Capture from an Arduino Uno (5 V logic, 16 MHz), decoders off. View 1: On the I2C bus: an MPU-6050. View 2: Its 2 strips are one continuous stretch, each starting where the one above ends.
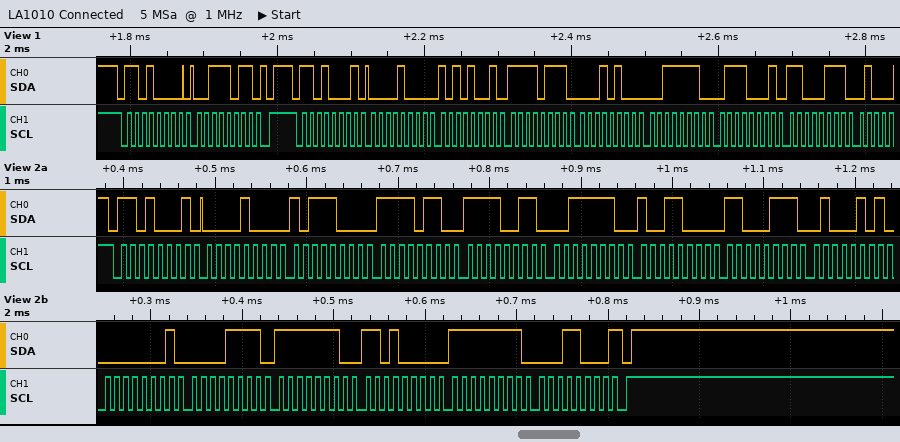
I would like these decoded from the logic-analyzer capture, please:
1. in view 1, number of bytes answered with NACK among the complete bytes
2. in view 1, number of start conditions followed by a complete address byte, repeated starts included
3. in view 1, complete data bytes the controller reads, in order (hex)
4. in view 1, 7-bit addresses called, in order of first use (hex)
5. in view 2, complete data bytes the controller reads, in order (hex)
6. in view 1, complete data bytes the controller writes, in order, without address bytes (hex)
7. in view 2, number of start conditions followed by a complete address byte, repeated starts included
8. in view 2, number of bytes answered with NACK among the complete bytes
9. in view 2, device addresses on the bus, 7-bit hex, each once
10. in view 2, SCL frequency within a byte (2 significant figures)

0
2
08 A9 F7 14 3E 71 C7
0x68
08 B8 F6 F3 3E 98 C7 45 01 0F FE D0 FF 18
3B
1
1
0x68
100 kHz
